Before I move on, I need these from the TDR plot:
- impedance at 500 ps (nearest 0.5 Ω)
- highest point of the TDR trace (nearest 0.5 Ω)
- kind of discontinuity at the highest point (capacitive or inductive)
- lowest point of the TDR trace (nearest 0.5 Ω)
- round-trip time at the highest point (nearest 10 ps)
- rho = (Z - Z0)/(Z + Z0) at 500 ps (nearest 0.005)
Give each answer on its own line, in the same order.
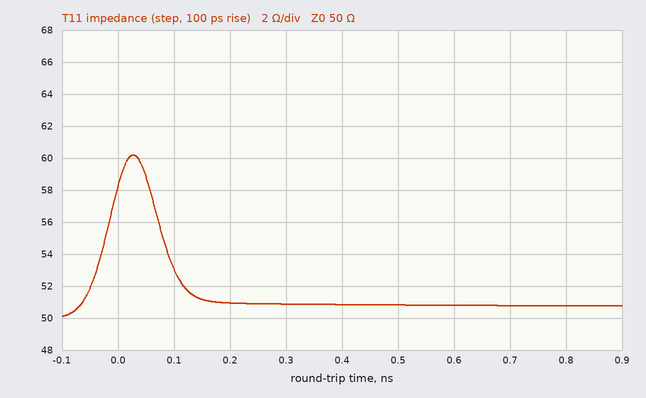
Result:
51.0 Ω
60.0 Ω
inductive
50.0 Ω
30 ps
+0.010
